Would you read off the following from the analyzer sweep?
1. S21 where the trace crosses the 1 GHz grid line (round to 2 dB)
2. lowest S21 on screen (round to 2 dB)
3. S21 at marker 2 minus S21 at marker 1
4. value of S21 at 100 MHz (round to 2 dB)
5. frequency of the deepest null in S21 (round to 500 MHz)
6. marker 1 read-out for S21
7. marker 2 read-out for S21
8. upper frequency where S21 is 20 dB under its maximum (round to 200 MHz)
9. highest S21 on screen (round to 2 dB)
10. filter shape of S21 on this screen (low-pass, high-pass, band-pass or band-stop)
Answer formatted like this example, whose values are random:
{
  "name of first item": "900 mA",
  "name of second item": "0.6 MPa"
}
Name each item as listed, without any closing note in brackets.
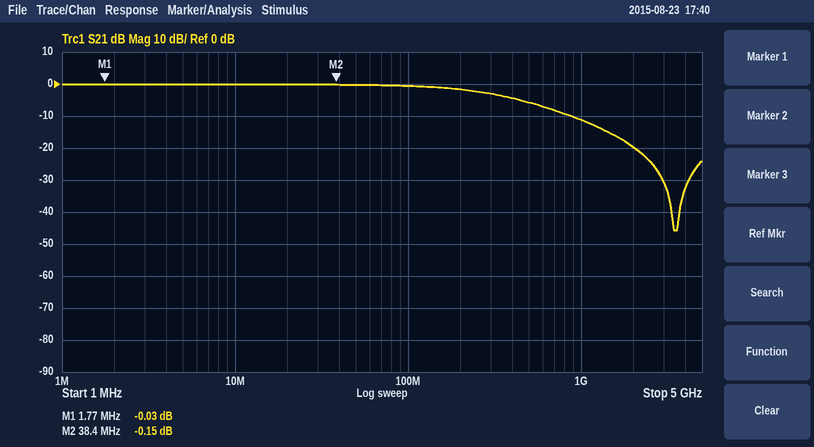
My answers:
{
  "S21 where the trace crosses the 1 GHz grid line": "-12 dB",
  "lowest S21 on screen": "-46 dB",
  "S21 at marker 2 minus S21 at marker 1": "-0.12 dB",
  "value of S21 at 100 MHz": "0 dB",
  "frequency of the deepest null in S21": "3.5 GHz",
  "marker 1 read-out for S21": "-0.03 dB",
  "marker 2 read-out for S21": "-0.15 dB",
  "upper frequency where S21 is 20 dB under its maximum": "2.0 GHz",
  "highest S21 on screen": "0 dB",
  "filter shape of S21 on this screen": "low-pass"
}
